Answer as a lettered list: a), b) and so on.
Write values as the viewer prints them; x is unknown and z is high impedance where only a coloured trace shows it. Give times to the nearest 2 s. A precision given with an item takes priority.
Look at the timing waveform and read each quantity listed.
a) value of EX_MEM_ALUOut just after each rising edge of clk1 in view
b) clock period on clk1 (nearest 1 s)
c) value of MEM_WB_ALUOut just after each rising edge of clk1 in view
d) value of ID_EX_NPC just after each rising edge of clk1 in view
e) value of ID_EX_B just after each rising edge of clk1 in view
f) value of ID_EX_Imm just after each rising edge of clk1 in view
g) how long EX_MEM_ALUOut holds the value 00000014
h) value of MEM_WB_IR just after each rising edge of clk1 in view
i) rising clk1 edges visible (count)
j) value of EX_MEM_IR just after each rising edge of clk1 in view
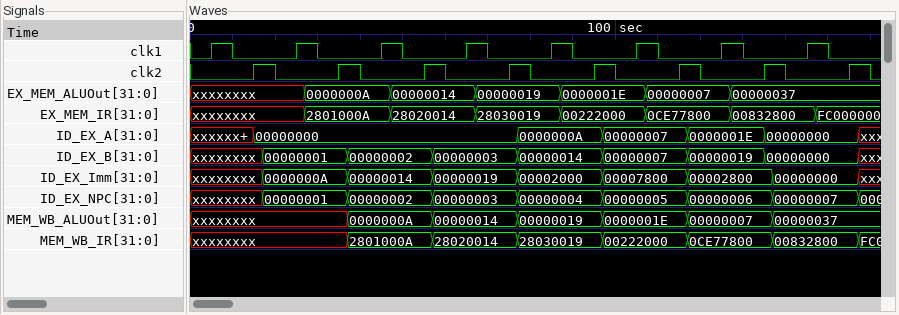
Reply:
a) xxxxxxxx, xxxxxxxx, 0000000A, 00000014, 00000019, 0000001E, 00000007, 00000037
b) 20 s
c) xxxxxxxx, xxxxxxxx, 0000000A, 00000014, 00000019, 0000001E, 00000007, 00000037
d) xxxxxxxx, 00000001, 00000002, 00000003, 00000004, 00000005, 00000006, 00000007
e) xxxxxxxx, 00000001, 00000002, 00000003, 00000014, 00000007, 00000019, 00000000
f) xxxxxxxx, 0000000A, 00000014, 00000019, 00002000, 00007800, 00002800, 00000000
g) 20 s
h) xxxxxxxx, xxxxxxxx, 2801000A, 28020014, 28030019, 00222000, 0CE77800, 00832800
i) 8
j) xxxxxxxx, xxxxxxxx, 2801000A, 28020014, 28030019, 00222000, 0CE77800, 00832800
